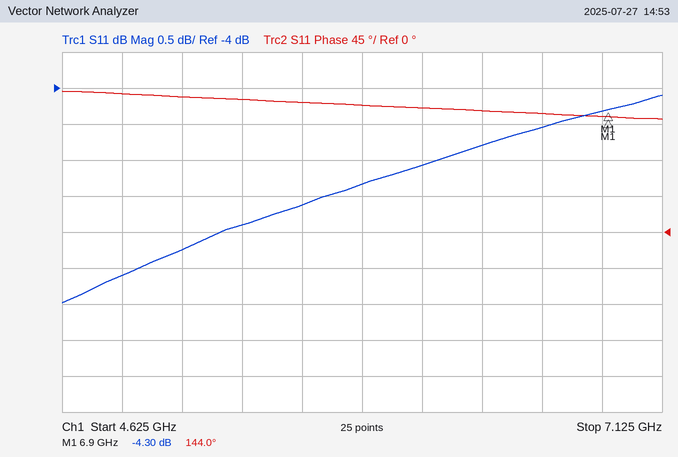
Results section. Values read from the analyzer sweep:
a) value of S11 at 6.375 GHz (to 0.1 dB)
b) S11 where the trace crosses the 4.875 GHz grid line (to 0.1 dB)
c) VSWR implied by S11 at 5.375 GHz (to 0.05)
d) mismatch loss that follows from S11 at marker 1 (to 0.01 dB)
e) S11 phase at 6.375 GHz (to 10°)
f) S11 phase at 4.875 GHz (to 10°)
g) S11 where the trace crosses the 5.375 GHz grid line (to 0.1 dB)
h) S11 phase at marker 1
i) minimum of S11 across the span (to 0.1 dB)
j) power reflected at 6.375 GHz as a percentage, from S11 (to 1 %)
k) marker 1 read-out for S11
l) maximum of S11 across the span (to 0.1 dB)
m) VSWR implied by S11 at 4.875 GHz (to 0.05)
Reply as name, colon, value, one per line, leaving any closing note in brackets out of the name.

value of S11 at 6.375 GHz: -4.8 dB
S11 where the trace crosses the 4.875 GHz grid line: -6.6 dB
VSWR implied by S11 at 5.375 GHz: 3.05
mismatch loss that follows from S11 at marker 1: 2.02 dB
S11 phase at 6.375 GHz: 150°
S11 phase at 4.875 GHz: 170°
S11 where the trace crosses the 5.375 GHz grid line: -5.9 dB
S11 phase at marker 1: 144.0°
minimum of S11 across the span: -7.0 dB
power reflected at 6.375 GHz as a percentage, from S11: 33 %
marker 1 read-out for S11: -4.30 dB
maximum of S11 across the span: -4.1 dB
VSWR implied by S11 at 4.875 GHz: 2.75
